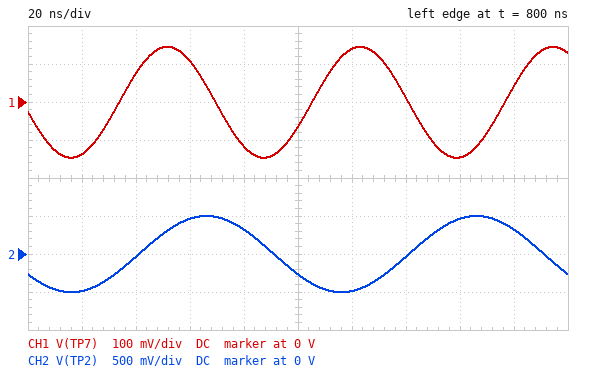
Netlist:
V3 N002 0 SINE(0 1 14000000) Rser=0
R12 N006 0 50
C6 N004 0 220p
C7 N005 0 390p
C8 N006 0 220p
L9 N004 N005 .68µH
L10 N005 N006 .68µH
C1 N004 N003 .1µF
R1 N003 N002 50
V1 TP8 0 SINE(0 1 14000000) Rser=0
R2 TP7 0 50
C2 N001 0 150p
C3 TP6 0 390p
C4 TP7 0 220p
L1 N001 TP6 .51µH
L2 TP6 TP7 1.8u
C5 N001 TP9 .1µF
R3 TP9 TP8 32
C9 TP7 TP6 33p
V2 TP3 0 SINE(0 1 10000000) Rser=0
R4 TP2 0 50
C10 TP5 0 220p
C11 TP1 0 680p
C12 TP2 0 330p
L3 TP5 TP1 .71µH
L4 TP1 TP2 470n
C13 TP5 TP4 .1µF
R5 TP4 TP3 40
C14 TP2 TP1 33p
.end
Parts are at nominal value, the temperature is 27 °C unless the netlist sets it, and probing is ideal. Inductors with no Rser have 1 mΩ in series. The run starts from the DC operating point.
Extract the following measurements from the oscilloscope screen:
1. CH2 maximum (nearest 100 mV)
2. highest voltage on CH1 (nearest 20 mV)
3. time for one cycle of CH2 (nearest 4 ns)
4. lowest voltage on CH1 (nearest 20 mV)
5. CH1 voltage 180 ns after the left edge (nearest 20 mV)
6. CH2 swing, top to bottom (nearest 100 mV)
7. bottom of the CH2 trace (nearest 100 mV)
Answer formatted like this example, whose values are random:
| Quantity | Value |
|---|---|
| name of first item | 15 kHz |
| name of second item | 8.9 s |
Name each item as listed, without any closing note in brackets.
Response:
| Quantity | Value |
|---|---|
| CH2 maximum | 500 mV |
| highest voltage on CH1 | 140 mV |
| time for one cycle of CH2 | 100 ns |
| lowest voltage on CH1 | -140 mV |
| CH1 voltage 180 ns after the left edge | 40 mV |
| CH2 swing, top to bottom | 1.0 V |
| bottom of the CH2 trace | -500 mV |
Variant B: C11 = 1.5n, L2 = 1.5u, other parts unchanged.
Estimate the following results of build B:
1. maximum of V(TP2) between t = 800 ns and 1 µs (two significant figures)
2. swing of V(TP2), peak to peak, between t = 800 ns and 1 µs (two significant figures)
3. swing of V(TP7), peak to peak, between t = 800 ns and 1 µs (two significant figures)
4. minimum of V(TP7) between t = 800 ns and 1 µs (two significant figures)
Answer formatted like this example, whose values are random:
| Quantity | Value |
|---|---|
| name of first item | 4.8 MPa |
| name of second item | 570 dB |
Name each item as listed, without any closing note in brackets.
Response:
| Quantity | Value |
|---|---|
| maximum of V(TP2) between t = 800 ns and 1 µs | 330 mV |
| swing of V(TP2), peak to peak, between t = 800 ns and 1 µs | 670 mV |
| swing of V(TP7), peak to peak, between t = 800 ns and 1 µs | 430 mV |
| minimum of V(TP7) between t = 800 ns and 1 µs | -210 mV |
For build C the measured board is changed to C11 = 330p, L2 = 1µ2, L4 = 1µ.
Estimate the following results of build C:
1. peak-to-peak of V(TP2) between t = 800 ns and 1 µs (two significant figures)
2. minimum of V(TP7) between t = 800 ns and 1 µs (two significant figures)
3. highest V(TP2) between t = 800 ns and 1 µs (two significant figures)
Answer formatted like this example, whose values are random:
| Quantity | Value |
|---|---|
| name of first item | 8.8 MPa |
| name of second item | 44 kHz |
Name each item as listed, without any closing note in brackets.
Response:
| Quantity | Value |
|---|---|
| peak-to-peak of V(TP2) between t = 800 ns and 1 µs | 950 mV |
| minimum of V(TP7) between t = 800 ns and 1 µs | -320 mV |
| highest V(TP2) between t = 800 ns and 1 µs | 470 mV |
